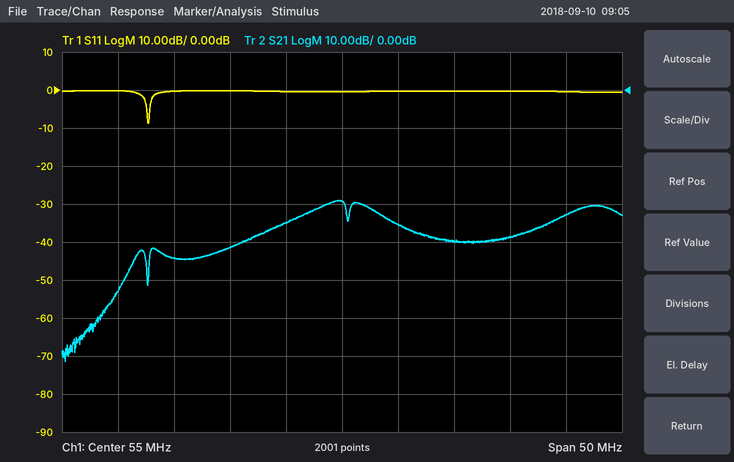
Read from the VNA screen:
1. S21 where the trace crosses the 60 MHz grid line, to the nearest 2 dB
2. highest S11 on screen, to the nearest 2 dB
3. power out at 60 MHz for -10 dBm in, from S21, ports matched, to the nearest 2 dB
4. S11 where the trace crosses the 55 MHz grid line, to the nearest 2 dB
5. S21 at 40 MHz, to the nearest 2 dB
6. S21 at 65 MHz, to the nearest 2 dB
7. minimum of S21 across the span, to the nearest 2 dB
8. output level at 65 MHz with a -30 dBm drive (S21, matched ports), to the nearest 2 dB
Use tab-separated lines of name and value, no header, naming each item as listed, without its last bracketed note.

S21 where the trace crosses the 60 MHz grid line, to the nearest 2 dB	-36 dB
highest S11 on screen, to the nearest 2 dB	0 dB
power out at 60 MHz for -10 dBm in, from S21, ports matched, to the nearest 2 dB	-46 dBm
S11 where the trace crosses the 55 MHz grid line, to the nearest 2 dB	0 dB
S21 at 40 MHz, to the nearest 2 dB	-44 dB
S21 at 65 MHz, to the nearest 2 dB	-40 dB
minimum of S21 across the span, to the nearest 2 dB	-72 dB
output level at 65 MHz with a -30 dBm drive (S21, matched ports), to the nearest 2 dB	-70 dBm
